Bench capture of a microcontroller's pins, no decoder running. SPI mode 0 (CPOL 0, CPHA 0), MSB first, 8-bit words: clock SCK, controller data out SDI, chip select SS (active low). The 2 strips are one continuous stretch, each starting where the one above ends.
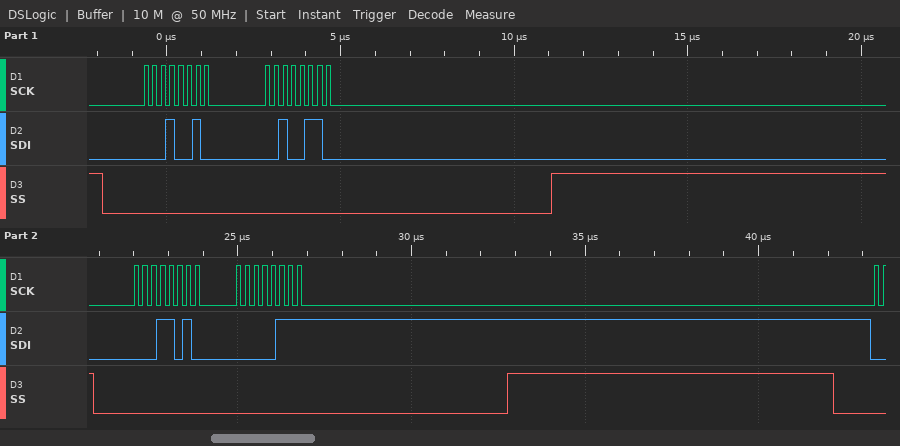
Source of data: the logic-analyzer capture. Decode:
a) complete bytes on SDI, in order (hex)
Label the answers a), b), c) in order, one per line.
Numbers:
a) 12 26 1A 07
